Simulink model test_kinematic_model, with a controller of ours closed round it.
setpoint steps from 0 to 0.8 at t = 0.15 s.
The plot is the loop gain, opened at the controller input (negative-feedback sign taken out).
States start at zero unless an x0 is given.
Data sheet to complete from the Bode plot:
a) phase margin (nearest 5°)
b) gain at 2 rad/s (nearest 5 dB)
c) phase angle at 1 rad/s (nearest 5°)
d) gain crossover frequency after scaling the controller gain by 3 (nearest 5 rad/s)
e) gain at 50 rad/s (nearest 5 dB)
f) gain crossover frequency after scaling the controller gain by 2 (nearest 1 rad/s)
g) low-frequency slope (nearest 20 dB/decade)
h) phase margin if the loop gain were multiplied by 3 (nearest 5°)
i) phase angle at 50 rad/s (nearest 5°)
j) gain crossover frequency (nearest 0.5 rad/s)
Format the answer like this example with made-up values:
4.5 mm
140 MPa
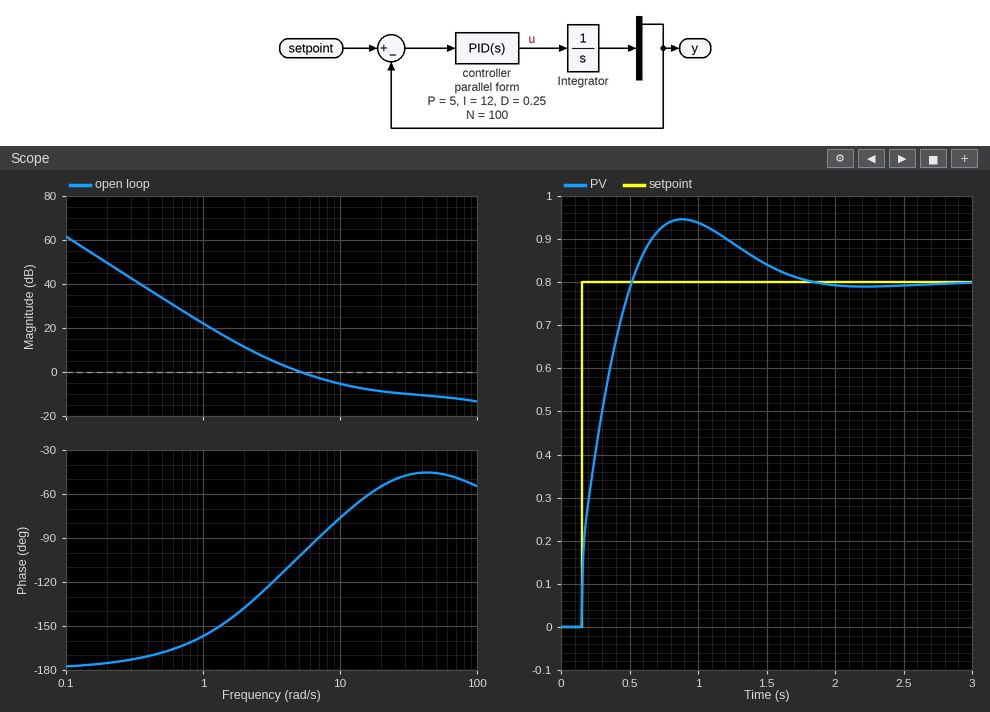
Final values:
80°
10 dB
-155°
25 rad/s
-10 dB
11 rad/s
-40 dB/decade
130°
-45°
5.0 rad/s
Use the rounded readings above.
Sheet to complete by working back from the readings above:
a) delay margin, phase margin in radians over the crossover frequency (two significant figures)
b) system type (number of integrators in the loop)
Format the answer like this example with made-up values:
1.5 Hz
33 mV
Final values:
0.28 s
2
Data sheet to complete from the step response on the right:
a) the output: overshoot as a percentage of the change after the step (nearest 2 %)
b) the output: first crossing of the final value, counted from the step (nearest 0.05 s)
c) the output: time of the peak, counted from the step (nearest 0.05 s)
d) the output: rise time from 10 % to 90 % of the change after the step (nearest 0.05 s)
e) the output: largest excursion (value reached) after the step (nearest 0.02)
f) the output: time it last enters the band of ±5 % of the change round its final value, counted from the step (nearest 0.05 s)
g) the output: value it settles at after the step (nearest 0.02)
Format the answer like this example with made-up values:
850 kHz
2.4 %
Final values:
18 %
0.35 s
0.75 s
0.30 s
0.94
1.35 s
0.80
